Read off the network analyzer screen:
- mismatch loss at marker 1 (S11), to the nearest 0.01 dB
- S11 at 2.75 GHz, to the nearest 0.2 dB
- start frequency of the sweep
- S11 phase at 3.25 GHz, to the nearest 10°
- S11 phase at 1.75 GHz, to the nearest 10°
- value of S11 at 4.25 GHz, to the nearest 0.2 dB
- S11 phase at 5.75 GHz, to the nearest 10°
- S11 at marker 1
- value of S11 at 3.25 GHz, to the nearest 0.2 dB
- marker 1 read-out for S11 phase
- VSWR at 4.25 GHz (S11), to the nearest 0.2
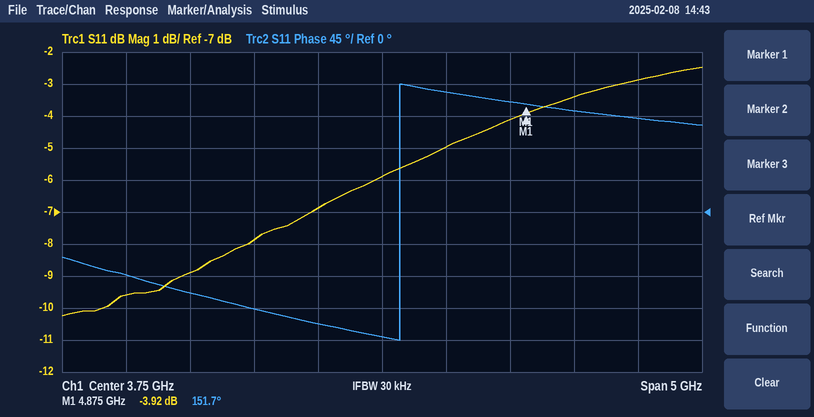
2.26 dB
-7.8 dB
1.25 GHz
-160°
-90°
-5.0 dB
130°
-3.92 dB
-6.8 dB
151.7°
3.6
